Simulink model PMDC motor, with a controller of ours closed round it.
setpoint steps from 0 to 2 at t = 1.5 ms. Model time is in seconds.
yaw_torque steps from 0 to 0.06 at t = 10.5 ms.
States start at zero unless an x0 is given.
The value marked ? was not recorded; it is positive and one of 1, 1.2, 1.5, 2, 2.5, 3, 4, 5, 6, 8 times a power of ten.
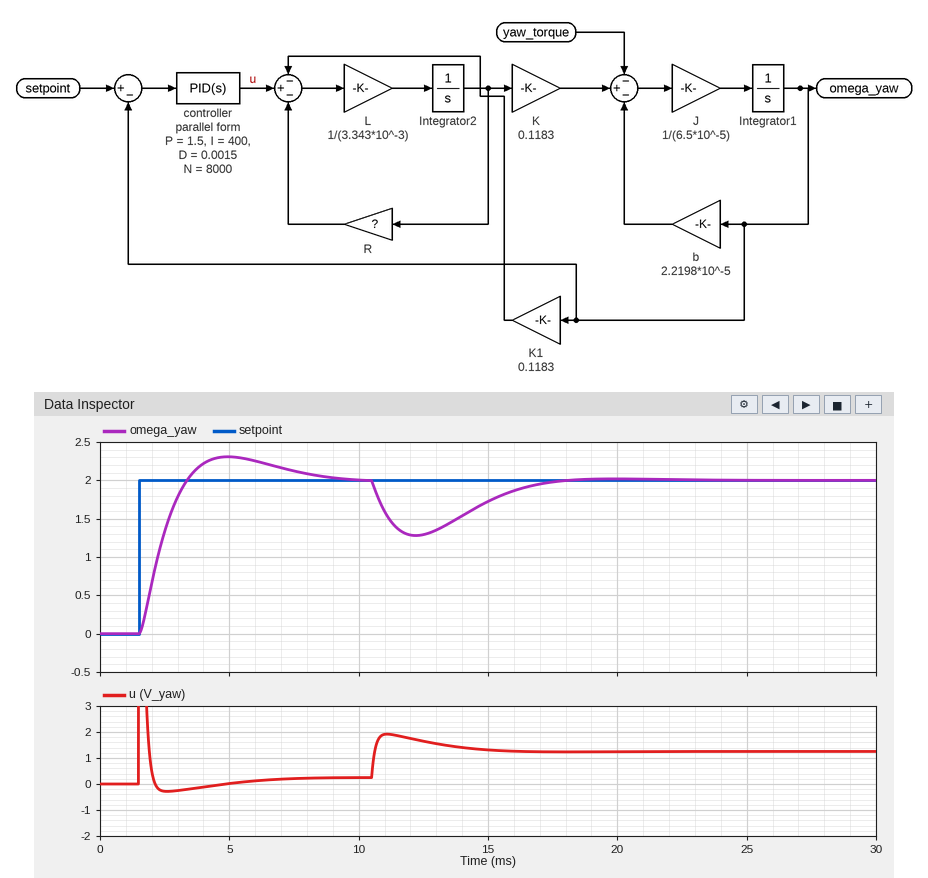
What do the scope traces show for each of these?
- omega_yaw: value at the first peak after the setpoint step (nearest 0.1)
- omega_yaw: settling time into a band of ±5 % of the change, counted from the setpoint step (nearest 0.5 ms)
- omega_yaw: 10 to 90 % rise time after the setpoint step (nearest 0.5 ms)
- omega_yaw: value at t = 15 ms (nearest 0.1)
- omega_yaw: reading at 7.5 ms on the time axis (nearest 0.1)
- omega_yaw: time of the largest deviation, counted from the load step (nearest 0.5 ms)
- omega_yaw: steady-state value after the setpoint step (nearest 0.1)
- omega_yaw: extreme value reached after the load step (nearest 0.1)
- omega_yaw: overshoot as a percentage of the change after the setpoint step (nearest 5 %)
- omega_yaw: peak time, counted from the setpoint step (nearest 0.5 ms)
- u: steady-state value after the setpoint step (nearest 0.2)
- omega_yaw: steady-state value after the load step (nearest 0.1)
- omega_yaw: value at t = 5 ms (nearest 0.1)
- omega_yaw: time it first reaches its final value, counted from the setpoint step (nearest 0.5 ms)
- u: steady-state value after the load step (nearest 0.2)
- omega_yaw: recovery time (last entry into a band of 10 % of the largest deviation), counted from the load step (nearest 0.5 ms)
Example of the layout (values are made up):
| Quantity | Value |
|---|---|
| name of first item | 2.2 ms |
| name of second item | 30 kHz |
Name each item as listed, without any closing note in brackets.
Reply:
| Quantity | Value |
|---|---|
| omega_yaw: value at the first peak after the setpoint step | 2.3 |
| omega_yaw: settling time into a band of ±5 % of the change, counted from the setpoint step | 6.5 ms |
| omega_yaw: 10 to 90 % rise time after the setpoint step | 1.5 ms |
| omega_yaw: value at t = 15 ms | 1.7 |
| omega_yaw: reading at 7.5 ms on the time axis | 2.1 |
| omega_yaw: time of the largest deviation, counted from the load step | 1.5 ms |
| omega_yaw: steady-state value after the setpoint step | 2.0 |
| omega_yaw: extreme value reached after the load step | 1.3 |
| omega_yaw: overshoot as a percentage of the change after the setpoint step | 15 % |
| omega_yaw: peak time, counted from the setpoint step | 3.5 ms |
| u: steady-state value after the setpoint step | 0.2 |
| omega_yaw: steady-state value after the load step | 2.0 |
| omega_yaw: value at t = 5 ms | 2.3 |
| omega_yaw: time it first reaches its final value, counted from the setpoint step | 2.0 ms |
| u: steady-state value after the load step | 1.2 |
| omega_yaw: recovery time (last entry into a band of 10 % of the largest deviation), counted from the load step | 6.0 ms |
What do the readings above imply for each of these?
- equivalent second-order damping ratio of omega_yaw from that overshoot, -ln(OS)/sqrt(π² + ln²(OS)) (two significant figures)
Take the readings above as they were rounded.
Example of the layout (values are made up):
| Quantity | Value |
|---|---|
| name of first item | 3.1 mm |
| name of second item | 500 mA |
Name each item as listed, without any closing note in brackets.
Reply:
| Quantity | Value |
|---|---|
| equivalent second-order damping ratio of omega_yaw from that overshoot, -ln(OS)/sqrt(π² + ln²(OS)) | 0.52 |
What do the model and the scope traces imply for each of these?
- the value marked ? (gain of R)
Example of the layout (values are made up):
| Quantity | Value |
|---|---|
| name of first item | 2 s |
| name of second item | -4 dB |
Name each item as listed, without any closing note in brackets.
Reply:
| Quantity | Value |
|---|---|
| the value marked ? | 2 |
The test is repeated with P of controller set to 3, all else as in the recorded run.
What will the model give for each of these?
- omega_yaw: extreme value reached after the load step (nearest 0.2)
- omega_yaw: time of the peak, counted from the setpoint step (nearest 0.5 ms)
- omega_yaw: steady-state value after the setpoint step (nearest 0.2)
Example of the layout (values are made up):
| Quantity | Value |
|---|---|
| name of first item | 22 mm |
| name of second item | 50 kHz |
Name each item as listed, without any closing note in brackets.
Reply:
| Quantity | Value |
|---|---|
| omega_yaw: extreme value reached after the load step | 1.4 |
| omega_yaw: time of the peak, counted from the setpoint step | 2.0 ms |
| omega_yaw: steady-state value after the setpoint step | 2.0 |
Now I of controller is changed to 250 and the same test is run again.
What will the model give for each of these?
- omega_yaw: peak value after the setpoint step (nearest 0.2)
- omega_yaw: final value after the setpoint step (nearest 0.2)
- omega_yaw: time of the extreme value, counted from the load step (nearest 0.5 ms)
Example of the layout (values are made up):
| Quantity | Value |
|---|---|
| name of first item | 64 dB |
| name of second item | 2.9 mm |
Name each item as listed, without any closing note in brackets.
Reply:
| Quantity | Value |
|---|---|
| omega_yaw: peak value after the setpoint step | 2.2 |
| omega_yaw: final value after the setpoint step | 2.0 |
| omega_yaw: time of the extreme value, counted from the load step | 2.0 ms |
